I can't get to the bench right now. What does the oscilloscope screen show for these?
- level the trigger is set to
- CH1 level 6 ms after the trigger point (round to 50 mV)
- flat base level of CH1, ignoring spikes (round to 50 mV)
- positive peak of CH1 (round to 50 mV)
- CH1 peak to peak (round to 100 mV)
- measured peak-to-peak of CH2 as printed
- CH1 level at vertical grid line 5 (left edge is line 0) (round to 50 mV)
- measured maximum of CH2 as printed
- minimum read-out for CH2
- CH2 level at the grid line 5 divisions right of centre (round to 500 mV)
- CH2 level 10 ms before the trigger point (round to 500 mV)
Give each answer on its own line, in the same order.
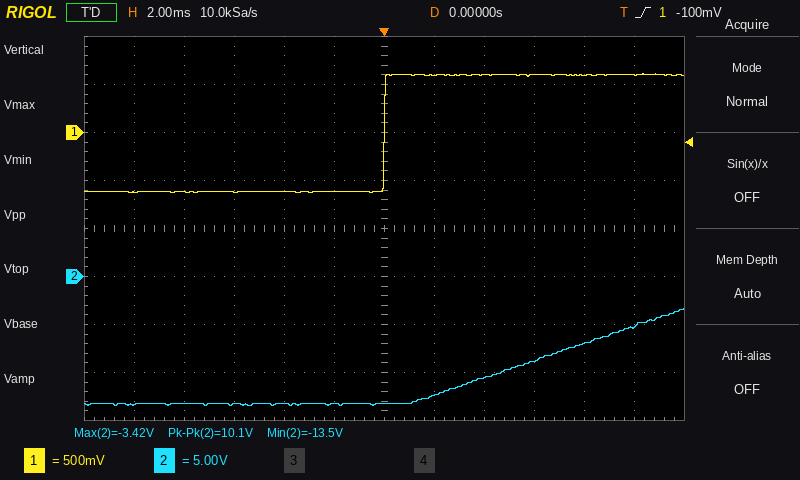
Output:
-100 mV
600 mV
-600 mV
600 mV
1.20 V
10.1 V
-600 mV
-3.42 V
-13.5 V
-5.0 V
-13.5 V
